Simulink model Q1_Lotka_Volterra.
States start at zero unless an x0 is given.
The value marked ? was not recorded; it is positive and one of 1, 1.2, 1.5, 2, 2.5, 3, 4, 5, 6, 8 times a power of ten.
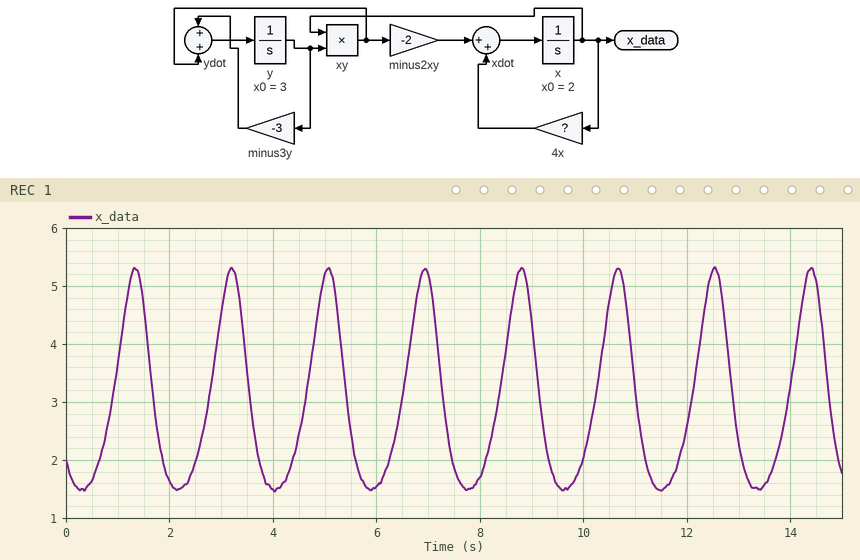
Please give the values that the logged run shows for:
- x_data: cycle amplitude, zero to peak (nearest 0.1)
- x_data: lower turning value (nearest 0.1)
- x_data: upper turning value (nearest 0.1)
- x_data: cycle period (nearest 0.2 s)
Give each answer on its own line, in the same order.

1.9
1.5
5.3
1.8 s
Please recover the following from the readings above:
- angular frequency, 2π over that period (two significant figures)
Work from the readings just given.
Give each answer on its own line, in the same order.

3.5 rad/s
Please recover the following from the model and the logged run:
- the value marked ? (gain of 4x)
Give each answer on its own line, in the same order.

4
